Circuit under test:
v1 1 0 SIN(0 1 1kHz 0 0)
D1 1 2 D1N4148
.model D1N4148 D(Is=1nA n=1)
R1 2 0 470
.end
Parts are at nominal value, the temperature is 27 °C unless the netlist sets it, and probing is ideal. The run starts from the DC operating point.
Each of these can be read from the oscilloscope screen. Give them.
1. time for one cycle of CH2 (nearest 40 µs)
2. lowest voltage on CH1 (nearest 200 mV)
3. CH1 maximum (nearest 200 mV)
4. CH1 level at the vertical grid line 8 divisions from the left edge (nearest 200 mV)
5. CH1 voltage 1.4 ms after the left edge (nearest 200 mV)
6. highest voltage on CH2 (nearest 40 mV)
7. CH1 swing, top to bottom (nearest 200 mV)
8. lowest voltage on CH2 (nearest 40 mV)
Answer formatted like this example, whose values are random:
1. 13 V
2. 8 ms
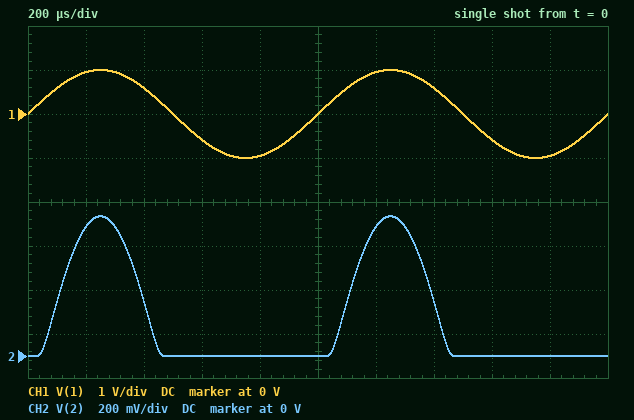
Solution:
1. 1.00 ms
2. -1.0 V
3. 1.0 V
4. -600 mV
5. 600 mV
6. 640 mV
7. 2.0 V
8. 0 V
